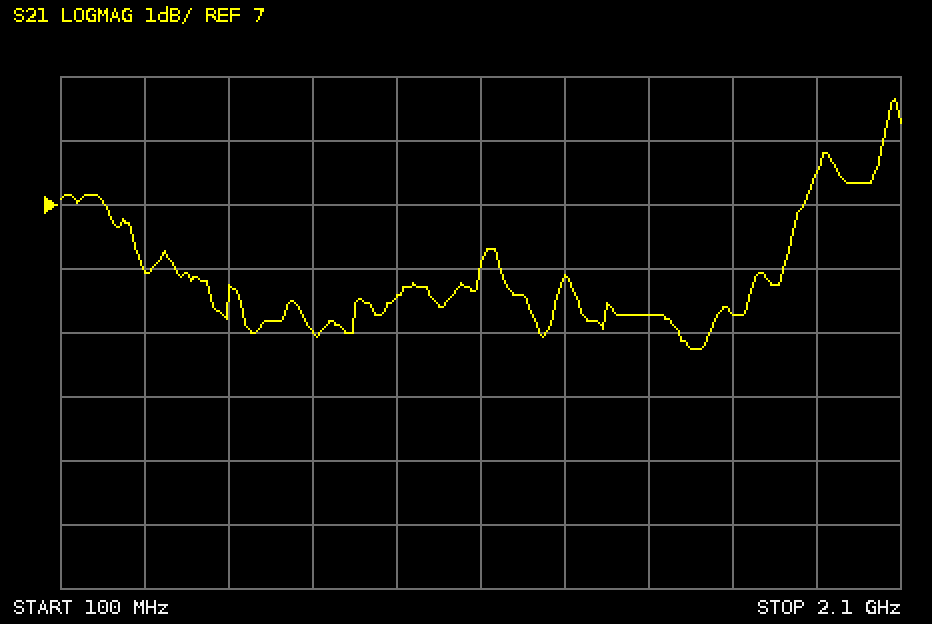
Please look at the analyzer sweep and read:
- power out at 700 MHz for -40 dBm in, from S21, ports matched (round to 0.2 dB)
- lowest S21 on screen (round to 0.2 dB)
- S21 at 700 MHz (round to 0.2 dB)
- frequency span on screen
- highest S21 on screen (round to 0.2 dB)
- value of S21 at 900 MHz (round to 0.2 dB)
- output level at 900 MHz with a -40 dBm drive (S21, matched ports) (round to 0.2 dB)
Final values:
-35.0 dBm
4.8 dB
5.0 dB
2 GHz
8.6 dB
5.6 dB
-34.4 dBm
